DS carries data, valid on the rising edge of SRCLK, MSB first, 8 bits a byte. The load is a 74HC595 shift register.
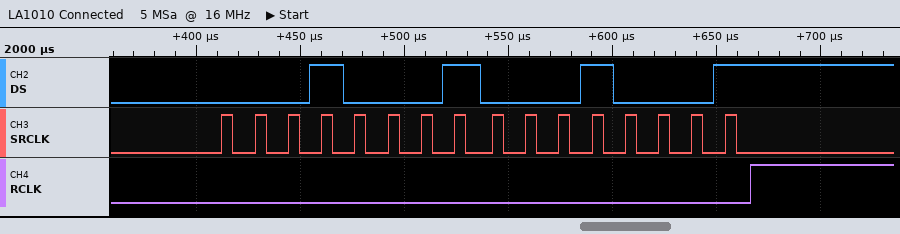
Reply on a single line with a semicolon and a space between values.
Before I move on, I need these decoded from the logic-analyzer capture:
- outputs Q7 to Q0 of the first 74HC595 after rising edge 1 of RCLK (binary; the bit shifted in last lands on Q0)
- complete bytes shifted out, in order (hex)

00010001; 11 11
